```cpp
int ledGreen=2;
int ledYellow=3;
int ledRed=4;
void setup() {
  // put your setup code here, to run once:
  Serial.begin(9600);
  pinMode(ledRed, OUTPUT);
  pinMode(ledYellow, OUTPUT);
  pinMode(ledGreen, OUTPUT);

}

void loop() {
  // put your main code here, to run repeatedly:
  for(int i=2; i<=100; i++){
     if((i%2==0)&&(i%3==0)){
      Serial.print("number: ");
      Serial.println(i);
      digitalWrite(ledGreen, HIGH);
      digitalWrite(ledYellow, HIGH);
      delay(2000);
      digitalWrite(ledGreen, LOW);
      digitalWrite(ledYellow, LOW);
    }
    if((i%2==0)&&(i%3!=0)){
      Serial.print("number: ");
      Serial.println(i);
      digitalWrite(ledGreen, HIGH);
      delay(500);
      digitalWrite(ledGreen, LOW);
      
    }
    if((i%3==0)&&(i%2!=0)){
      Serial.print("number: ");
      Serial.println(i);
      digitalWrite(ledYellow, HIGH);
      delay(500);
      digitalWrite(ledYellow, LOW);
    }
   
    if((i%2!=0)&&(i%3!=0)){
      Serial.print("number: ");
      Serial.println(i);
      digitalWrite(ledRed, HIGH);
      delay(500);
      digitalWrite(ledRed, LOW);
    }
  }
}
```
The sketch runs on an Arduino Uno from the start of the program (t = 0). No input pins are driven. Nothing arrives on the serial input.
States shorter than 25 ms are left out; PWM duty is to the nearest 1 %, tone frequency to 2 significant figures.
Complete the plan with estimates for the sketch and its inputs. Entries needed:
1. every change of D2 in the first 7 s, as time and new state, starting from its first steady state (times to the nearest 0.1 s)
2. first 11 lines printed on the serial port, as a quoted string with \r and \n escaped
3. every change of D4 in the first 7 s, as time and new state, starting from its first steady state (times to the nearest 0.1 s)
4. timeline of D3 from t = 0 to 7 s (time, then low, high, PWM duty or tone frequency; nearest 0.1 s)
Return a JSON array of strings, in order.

["0 s high; 0.5 s low; 1 s high; 1.5 s low; 2 s high; 4 s low; 4.5 s high; 5 s low; 5.5 s high; 6 s low; 6.5 s high", "\"number: 2\\r\\nnumber: 3\\r\\nnumber: 4\\r\\nnumber: 5\\r\\nnumber: 6\\r\\nnumber: 7\\r\\nnumber: 8\\r\\nnumber: 9\\r\\nnumber: 10\\r\\nnumber: 11\\r\\nnumber: 12\\r\\n\"", "0 s low; 1.5 s high; 2 s low; 4 s high; 4.5 s low; 6 s high; 6.5 s low", "0 s low; 0.5 s high; 1 s low; 2 s high; 4 s low; 5 s high; 5.5 s low; 6.5 s high"]
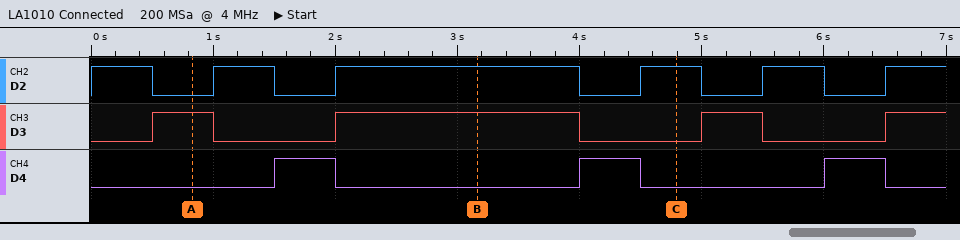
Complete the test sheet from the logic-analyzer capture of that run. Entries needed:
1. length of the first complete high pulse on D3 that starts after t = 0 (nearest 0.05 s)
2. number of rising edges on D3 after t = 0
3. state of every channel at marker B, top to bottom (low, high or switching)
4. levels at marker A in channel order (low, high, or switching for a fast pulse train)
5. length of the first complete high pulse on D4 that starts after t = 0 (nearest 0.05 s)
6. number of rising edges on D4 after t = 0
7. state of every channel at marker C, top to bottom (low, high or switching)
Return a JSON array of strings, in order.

["0.50 s", "4", "D2 high, D3 high, D4 low", "D2 low, D3 high, D4 low", "0.50 s", "3", "D2 high, D3 low, D4 low"]
